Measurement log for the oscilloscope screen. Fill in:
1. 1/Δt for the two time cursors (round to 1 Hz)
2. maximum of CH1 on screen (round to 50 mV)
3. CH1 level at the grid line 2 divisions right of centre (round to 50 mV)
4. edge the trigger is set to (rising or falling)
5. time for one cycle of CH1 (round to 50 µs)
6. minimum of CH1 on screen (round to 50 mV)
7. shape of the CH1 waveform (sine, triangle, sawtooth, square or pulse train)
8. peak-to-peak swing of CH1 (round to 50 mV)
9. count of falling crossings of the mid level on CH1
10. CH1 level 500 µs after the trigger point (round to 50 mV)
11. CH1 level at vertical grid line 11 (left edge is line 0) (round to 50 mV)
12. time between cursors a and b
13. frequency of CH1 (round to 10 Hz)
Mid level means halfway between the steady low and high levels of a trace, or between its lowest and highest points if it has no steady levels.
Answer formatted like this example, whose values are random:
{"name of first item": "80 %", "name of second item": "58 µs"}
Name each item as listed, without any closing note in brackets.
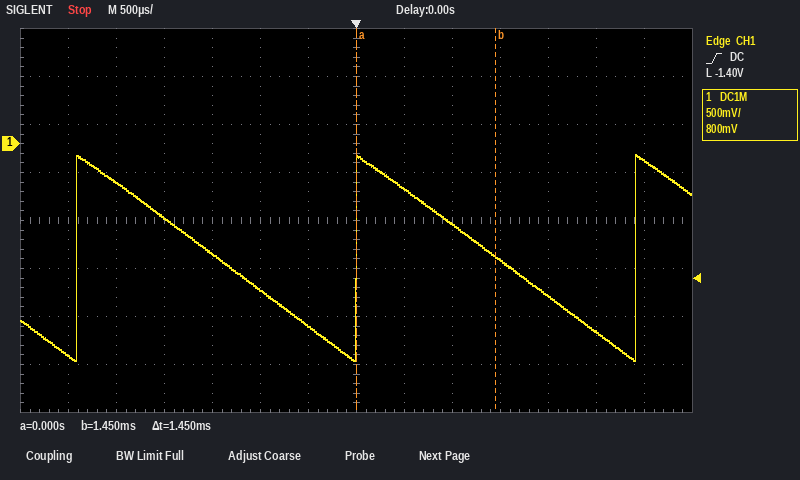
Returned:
{"1/Δt for the two time cursors": "690 Hz", "maximum of CH1 on screen": "-100 mV", "CH1 level at the grid line 2 divisions right of centre": "-850 mV", "edge the trigger is set to": "rising", "time for one cycle of CH1": "2.90 ms", "minimum of CH1 on screen": "-2.25 V", "shape of the CH1 waveform": "sawtooth", "peak-to-peak swing of CH1": "2.15 V", "count of falling crossings of the mid level on CH1": "2", "CH1 level 500 µs after the trigger point": "-450 mV", "CH1 level at vertical grid line 11 (left edge is line 0)": "-1.60 V", "time between cursors a and b": "1.45 ms", "frequency of CH1": "340 Hz"}
